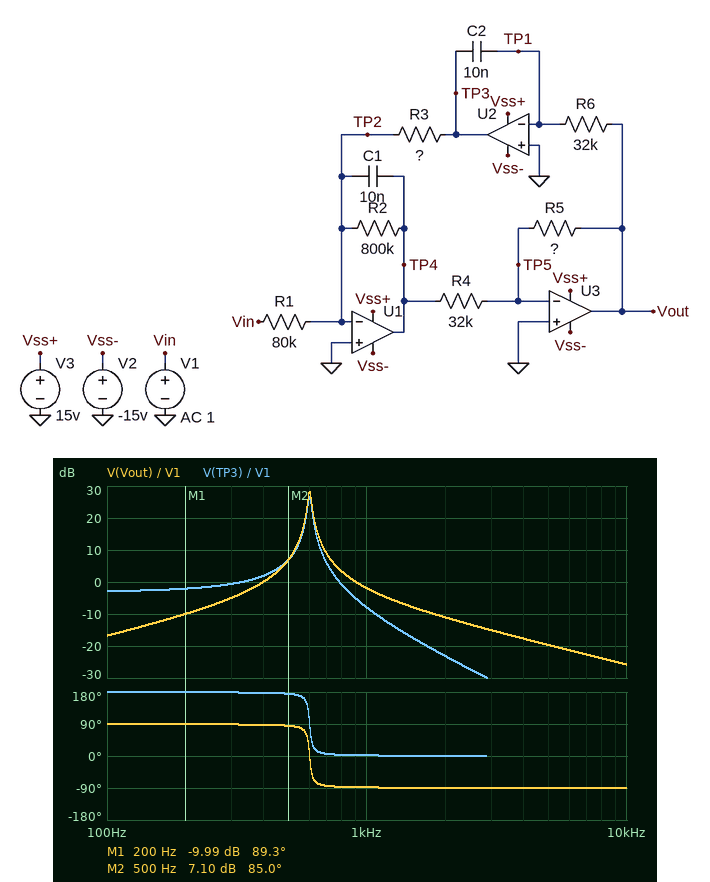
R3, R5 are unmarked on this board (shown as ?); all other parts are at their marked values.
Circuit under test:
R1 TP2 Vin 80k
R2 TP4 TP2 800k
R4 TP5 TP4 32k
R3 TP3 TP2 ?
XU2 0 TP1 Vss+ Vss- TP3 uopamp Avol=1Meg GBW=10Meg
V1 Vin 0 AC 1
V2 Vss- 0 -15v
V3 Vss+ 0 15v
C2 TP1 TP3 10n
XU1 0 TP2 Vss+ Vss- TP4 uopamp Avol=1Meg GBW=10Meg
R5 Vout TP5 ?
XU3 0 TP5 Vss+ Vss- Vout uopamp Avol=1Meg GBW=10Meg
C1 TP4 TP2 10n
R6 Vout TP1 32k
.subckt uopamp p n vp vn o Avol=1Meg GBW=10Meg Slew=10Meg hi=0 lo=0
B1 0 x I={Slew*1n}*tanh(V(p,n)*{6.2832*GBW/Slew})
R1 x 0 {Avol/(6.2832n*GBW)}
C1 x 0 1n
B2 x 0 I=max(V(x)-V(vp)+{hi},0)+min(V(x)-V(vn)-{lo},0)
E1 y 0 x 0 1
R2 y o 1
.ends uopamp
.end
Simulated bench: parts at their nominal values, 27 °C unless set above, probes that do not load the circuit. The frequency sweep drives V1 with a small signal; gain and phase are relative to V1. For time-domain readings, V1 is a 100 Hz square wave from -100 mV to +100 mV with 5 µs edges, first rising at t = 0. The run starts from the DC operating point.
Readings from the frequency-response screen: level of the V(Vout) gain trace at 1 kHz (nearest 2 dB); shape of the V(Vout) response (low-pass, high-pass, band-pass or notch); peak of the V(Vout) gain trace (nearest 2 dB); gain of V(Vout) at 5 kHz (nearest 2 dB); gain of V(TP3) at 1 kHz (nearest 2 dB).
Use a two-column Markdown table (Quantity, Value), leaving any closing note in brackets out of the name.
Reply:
| Quantity | Value |
|---|---|
| level of the V(Vout) gain trace at 1 kHz | -2 dB |
| shape of the V(Vout) response | band-pass |
| peak of the V(Vout) gain trace | 28 dB |
| gain of V(Vout) at 5 kHz | -20 dB |
| gain of V(TP3) at 1 kHz | -8 dB |
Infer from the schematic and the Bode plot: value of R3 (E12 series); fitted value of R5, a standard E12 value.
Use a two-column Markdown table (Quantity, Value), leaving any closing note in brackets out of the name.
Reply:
| Quantity | Value |
|---|---|
| value of R3 | 56 kΩ |
| fitted value of R5, a standard E12 value | 82 kΩ |
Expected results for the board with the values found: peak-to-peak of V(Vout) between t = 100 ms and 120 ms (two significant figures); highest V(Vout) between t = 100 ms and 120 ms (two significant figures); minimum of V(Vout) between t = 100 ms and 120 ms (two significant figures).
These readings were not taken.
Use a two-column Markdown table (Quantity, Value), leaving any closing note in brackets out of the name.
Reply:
| Quantity | Value |
|---|---|
| peak-to-peak of V(Vout) between t = 100 ms and 120 ms | 190 mV |
| highest V(Vout) between t = 100 ms and 120 ms | 95 mV |
| minimum of V(Vout) between t = 100 ms and 120 ms | -95 mV |
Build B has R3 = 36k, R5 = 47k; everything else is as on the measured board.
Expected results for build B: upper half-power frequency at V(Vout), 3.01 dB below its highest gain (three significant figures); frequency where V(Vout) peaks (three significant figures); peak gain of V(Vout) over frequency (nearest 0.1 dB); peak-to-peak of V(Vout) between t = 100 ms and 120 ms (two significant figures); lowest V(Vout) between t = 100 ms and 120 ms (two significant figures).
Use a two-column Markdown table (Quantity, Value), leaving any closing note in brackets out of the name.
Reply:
| Quantity | Value |
|---|---|
| upper half-power frequency at V(Vout), 3.01 dB below its highest gain | 578 Hz |
| frequency where V(Vout) peaks | 568 Hz |
| peak gain of V(Vout) over frequency | 23.4 dB |
| peak-to-peak of V(Vout) between t = 100 ms and 120 ms | 130 mV |
| lowest V(Vout) between t = 100 ms and 120 ms | -66 mV |
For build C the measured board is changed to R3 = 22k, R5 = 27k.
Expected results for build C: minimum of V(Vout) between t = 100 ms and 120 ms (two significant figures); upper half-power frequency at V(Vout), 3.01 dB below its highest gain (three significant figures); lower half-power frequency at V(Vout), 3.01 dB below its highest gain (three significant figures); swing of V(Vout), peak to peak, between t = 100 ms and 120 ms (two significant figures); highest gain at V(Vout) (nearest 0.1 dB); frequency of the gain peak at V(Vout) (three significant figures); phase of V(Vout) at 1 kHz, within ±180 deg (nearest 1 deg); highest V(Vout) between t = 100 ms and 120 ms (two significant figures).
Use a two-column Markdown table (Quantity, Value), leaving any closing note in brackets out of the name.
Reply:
| Quantity | Value |
|---|---|
| minimum of V(Vout) between t = 100 ms and 120 ms | -48 mV |
| upper half-power frequency at V(Vout), 3.01 dB below its highest gain | 561 Hz |
| lower half-power frequency at V(Vout), 3.01 dB below its highest gain | 541 Hz |
| swing of V(Vout), peak to peak, between t = 100 ms and 120 ms | 96 mV |
| highest gain at V(Vout) | 18.6 dB |
| frequency of the gain peak at V(Vout) | 551 Hz |
| phase of V(Vout) at 1 kHz, within ±180 deg | -88 deg |
| highest V(Vout) between t = 100 ms and 120 ms | 48 mV |
